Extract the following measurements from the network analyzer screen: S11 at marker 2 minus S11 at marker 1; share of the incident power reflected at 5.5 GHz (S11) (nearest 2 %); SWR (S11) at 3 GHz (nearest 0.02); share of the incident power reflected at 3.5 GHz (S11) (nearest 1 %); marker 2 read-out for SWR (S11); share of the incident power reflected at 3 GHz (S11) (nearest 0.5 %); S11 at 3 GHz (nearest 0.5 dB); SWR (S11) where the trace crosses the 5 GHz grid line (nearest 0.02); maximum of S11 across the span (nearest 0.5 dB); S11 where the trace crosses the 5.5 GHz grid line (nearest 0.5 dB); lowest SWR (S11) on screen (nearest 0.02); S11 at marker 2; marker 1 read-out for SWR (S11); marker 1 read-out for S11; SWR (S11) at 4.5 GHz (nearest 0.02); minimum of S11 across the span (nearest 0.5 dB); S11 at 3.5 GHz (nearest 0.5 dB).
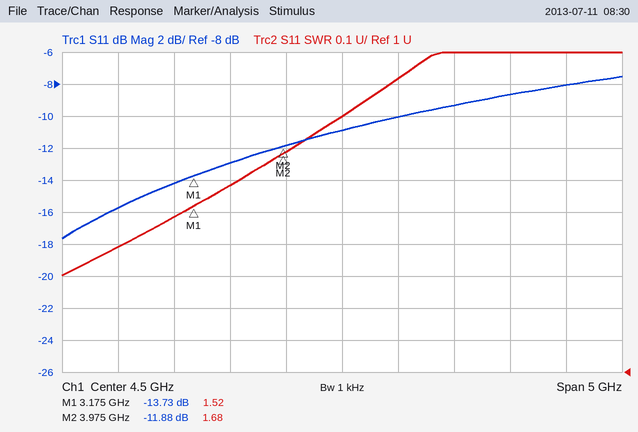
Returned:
1.85 dB
12 %
1.48
5 %
1.68
4.0 %
-14.0 dB
1.92
-7.5 dB
-9.5 dB
1.30
-11.88 dB
1.52
-13.73 dB
1.80
-17.5 dB
-13.0 dB
